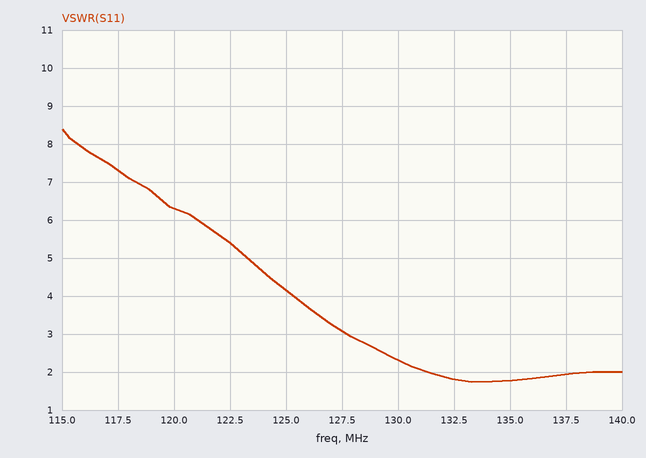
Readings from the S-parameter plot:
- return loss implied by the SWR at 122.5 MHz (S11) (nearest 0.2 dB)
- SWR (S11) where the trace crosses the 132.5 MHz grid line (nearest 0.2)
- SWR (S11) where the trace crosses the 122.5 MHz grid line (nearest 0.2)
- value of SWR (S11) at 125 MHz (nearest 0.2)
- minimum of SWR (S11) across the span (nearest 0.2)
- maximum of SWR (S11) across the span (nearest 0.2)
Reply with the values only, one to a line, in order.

3.2 dB
1.8
5.4
4.2
1.8
8.4
